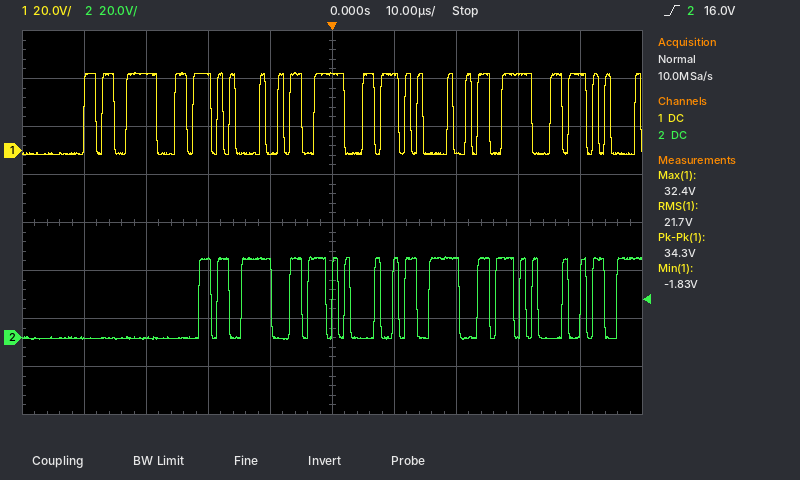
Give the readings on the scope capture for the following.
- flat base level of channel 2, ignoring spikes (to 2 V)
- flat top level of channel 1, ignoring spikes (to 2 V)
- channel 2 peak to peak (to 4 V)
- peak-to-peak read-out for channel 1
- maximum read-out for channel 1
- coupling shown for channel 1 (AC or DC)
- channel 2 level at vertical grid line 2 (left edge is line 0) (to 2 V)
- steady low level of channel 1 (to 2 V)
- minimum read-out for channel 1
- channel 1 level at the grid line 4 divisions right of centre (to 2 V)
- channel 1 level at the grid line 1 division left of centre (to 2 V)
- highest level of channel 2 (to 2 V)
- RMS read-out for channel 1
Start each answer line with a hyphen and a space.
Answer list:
- 0 V
- 32 V
- 36 V
- 34.3 V
- 32.4 V
- DC
- 0 V
- -2 V
- -1.83 V
- 32 V
- -2 V
- 34 V
- 21.7 V
